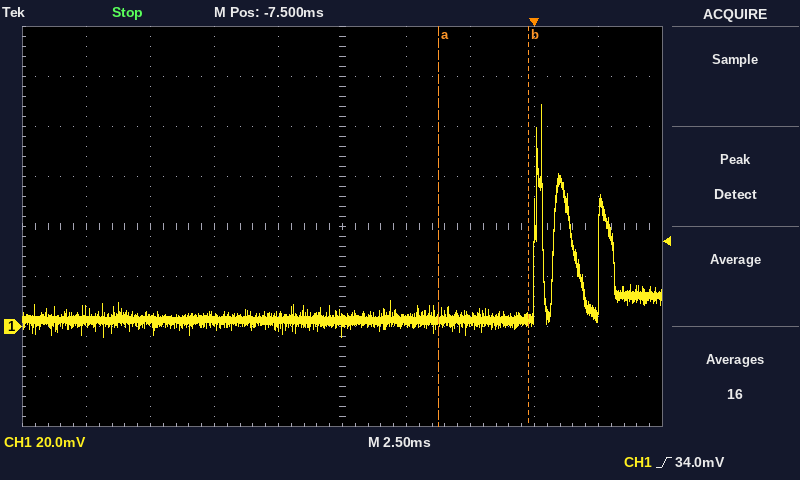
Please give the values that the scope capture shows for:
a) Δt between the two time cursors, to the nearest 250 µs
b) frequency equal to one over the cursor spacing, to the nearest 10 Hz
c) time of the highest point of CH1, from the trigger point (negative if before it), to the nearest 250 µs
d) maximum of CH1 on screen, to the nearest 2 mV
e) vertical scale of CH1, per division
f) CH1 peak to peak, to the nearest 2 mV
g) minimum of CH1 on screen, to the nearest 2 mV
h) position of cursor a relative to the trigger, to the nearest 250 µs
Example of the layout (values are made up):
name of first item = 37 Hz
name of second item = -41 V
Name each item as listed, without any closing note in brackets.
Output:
Δt between the two time cursors, to the nearest 250 µs = 3.50 ms
frequency equal to one over the cursor spacing, to the nearest 10 Hz = 290 Hz
time of the highest point of CH1, from the trigger point (negative if before it), to the nearest 250 µs = +250 µs
maximum of CH1 on screen, to the nearest 2 mV = 88 mV
vertical scale of CH1, per division = 20 mV
CH1 peak to peak, to the nearest 2 mV = 92 mV
minimum of CH1 on screen, to the nearest 2 mV = -4 mV
position of cursor a relative to the trigger, to the nearest 250 µs = -3.75 ms
